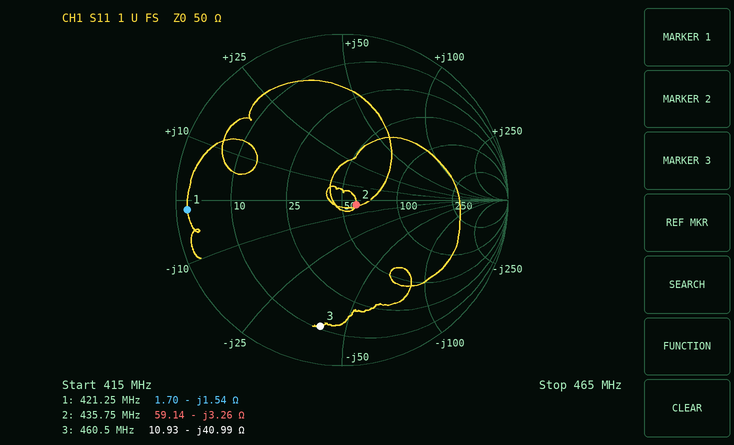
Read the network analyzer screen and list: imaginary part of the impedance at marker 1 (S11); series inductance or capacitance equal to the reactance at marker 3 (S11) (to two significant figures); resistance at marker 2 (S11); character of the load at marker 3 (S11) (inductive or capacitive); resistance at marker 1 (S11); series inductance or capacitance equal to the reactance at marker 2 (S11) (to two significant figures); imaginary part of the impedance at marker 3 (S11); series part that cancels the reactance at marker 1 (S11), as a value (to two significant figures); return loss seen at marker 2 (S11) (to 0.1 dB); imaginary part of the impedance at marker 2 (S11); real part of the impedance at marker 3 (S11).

-1.54 Ω
8.4 pF
59.14 Ω
capacitive
1.70 Ω
110 pF
-40.99 Ω
580 pH
21.0 dB
-3.26 Ω
10.93 Ω
